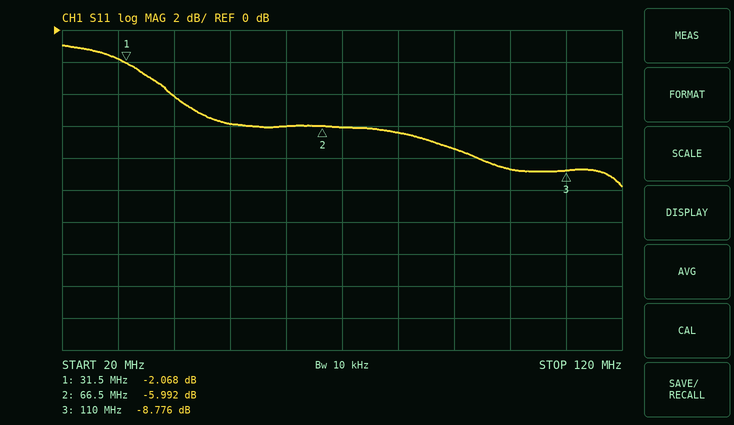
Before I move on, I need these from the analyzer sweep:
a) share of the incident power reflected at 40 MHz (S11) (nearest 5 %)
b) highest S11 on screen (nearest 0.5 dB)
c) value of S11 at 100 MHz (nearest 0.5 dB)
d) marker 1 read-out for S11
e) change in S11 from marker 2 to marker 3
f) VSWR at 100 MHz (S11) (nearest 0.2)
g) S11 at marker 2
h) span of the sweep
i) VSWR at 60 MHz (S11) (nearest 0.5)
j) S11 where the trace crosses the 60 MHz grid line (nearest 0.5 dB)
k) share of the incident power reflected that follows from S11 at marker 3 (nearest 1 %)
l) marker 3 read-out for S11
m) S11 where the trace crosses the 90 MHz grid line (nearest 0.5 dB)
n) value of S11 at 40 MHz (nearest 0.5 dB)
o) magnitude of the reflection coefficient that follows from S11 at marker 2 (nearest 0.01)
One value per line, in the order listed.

40 %
-1.0 dB
-8.5 dB
-2.068 dB
-2.784 dB
2.2
-5.992 dB
100 MHz
3.0
-6.0 dB
13 %
-8.776 dB
-7.5 dB
-4.0 dB
0.50
